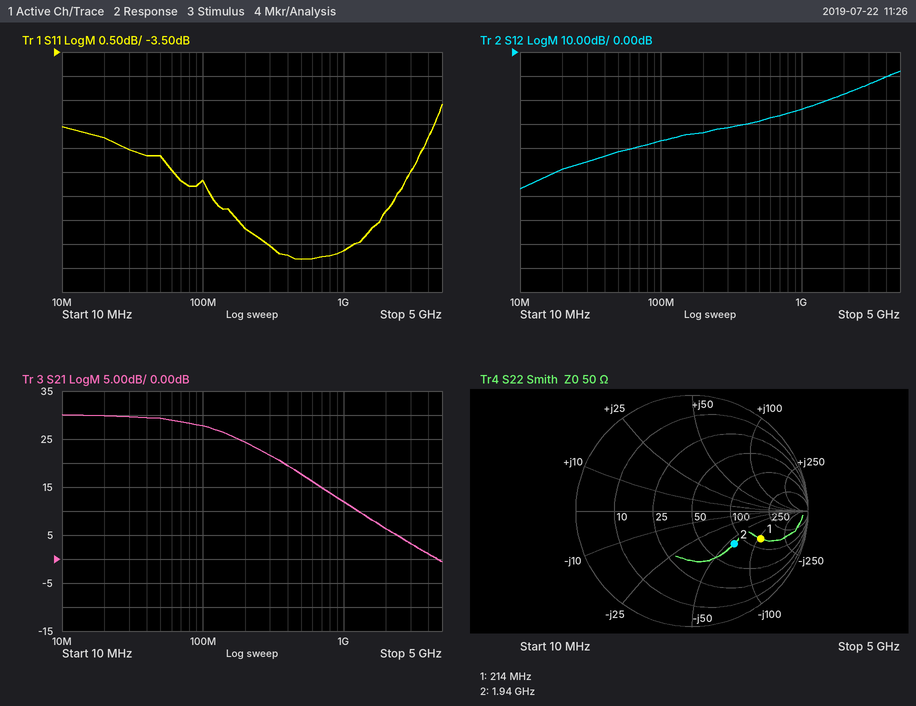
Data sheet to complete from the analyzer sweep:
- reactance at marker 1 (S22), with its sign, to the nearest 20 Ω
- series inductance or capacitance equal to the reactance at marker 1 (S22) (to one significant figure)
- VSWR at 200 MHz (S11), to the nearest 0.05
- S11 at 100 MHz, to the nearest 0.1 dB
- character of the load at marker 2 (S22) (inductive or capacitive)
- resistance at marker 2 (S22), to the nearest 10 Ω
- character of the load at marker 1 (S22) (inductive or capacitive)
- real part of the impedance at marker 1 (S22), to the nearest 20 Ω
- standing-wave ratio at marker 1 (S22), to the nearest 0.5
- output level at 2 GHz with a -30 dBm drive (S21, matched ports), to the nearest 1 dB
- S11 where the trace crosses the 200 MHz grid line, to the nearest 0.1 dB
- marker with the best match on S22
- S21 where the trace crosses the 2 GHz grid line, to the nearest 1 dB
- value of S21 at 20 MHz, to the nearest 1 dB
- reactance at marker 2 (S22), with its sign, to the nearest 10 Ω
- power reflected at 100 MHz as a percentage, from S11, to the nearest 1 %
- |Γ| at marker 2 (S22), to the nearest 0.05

-100 Ω
7 pF
2.55
-6.2 dB
capacitive
80 Ω
capacitive
140 Ω
4.5
-24 dBm
-7.2 dB
marker 2
6 dB
30 dB
-60 Ω
24 %
0.45
